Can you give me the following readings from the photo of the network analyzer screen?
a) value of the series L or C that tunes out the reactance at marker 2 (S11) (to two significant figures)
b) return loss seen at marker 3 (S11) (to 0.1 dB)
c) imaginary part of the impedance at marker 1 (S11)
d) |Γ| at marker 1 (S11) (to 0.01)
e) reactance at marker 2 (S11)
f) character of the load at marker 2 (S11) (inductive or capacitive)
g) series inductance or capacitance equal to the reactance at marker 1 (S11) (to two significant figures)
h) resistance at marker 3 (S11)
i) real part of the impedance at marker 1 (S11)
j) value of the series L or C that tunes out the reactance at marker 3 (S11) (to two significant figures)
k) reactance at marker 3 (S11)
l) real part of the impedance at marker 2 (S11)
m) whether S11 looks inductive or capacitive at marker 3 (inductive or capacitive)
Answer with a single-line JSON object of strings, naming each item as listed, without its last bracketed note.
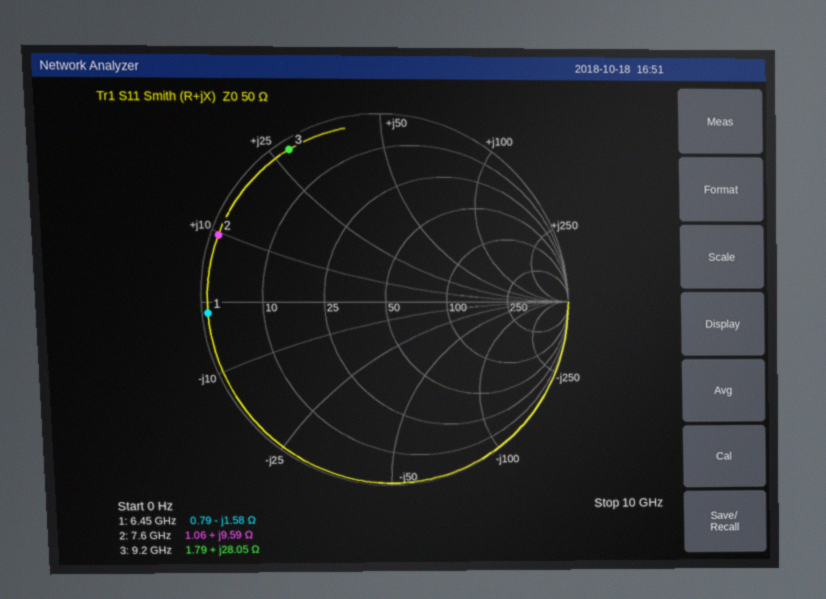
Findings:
{"value of the series L or C that tunes out the reactance at marker 2 (S11)": "2.2 pF", "return loss seen at marker 3 (S11)": "0.5 dB", "imaginary part of the impedance at marker 1": "-1.58 Ω", "|Γ| at marker 1 (S11)": "0.97", "reactance at marker 2": "+9.59 Ω", "character of the load at marker 2 (S11)": "inductive", "series inductance or capacitance equal to the reactance at marker 1 (S11)": "16 pF", "resistance at marker 3": "1.79 Ω", "real part of the impedance at marker 1": "0.79 Ω", "value of the series L or C that tunes out the reactance at marker 3 (S11)": "620 fF", "reactance at marker 3": "+28.05 Ω", "real part of the impedance at marker 2": "1.06 Ω", "whether S11 looks inductive or capacitive at marker 3": "inductive"}
